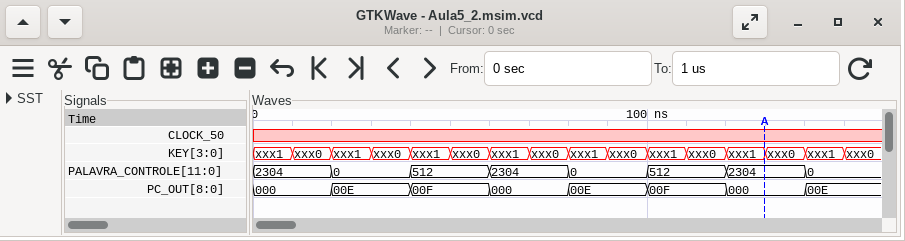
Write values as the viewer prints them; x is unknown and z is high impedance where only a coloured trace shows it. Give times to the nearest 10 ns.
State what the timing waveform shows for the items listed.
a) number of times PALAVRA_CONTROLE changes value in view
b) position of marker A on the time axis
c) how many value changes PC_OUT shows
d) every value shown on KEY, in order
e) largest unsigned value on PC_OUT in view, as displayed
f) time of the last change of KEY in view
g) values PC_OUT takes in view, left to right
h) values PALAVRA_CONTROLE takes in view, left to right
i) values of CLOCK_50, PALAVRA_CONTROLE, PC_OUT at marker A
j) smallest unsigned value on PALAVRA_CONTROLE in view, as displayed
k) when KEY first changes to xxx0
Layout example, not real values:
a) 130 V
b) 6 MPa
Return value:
a) 7
b) 130 ns
c) 7
d) xxx1, xxx0, xxx1, xxx0, xxx1, xxx0, xxx1, xxx0, xxx1, xxx0, xxx1, xxx0, xxx1, xxx0, xxx1, xxx0
e) 00F
f) 150 ns
g) 000, 00E, 00F, 000, 00E, 00F, 000, 00E
h) 2304, 0, 512, 2304, 0, 512, 2304, 0
i) CLOCK_50=x, PALAVRA_CONTROLE=2304, PC_OUT=000
j) 0
k) 10 ns
